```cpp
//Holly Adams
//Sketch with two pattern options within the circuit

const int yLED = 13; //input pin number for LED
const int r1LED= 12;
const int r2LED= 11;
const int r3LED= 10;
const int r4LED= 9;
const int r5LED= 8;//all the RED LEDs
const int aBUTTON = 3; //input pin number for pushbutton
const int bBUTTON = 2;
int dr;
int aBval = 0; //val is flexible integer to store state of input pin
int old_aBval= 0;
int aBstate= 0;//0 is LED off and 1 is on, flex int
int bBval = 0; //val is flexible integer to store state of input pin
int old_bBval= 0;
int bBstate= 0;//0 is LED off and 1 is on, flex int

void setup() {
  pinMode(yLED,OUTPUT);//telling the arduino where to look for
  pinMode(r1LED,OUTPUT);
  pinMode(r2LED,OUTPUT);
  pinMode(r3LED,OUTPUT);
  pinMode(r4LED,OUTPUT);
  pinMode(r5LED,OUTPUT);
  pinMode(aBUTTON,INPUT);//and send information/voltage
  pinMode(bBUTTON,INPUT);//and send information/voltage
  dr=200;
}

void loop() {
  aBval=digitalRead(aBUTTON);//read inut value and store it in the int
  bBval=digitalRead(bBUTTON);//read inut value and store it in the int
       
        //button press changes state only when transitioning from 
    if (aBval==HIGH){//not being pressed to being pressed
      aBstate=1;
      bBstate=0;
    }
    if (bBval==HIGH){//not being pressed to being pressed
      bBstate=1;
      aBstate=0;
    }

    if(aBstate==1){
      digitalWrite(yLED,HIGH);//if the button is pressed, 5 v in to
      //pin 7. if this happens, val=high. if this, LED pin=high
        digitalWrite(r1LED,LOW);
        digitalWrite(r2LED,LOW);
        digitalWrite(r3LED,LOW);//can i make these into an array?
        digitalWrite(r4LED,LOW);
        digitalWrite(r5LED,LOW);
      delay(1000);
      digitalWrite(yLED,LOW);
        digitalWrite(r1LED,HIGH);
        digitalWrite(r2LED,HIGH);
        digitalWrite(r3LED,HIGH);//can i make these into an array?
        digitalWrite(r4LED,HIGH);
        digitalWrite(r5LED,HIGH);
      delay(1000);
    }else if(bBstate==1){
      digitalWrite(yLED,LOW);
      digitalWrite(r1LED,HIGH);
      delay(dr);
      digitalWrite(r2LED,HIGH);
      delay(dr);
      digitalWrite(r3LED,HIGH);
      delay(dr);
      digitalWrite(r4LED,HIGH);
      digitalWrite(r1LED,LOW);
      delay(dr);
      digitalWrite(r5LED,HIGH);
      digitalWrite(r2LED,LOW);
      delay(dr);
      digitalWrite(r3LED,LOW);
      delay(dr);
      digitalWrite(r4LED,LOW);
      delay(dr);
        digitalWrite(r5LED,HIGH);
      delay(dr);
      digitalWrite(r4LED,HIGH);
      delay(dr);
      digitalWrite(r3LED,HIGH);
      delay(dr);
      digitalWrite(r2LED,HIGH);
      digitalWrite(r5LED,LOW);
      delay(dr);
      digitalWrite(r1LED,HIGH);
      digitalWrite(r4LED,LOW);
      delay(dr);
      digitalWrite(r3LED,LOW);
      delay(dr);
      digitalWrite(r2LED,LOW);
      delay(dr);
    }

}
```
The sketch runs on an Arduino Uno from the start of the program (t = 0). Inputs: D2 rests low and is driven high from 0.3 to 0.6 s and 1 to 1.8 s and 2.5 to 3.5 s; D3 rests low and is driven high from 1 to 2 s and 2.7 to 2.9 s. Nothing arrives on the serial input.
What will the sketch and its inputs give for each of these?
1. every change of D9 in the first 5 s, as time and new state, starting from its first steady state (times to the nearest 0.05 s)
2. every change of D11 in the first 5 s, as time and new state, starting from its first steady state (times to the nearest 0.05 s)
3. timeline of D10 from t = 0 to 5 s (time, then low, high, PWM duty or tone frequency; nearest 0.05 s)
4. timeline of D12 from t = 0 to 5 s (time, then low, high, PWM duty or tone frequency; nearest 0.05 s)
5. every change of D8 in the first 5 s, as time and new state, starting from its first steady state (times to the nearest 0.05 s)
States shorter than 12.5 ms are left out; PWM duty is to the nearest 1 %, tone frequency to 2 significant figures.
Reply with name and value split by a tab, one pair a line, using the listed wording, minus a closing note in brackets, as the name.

every change of D9 in the first 5 s, as time and new state, starting from its first steady state	0 s low; 0.9 s high; 1.5 s low; 1.9 s high; 2.5 s low; 3.7 s high; 4.3 s low; 4.7 s high
every change of D11 in the first 5 s, as time and new state, starting from its first steady state	0 s low; 0.5 s high; 1.1 s low; 2.3 s high; 2.9 s low; 3.3 s high; 3.9 s low
timeline of D10 from t = 0 to 5 s	0 s low; 0.7 s high; 1.3 s low; 2.1 s high; 2.7 s low; 3.5 s high; 4.1 s low; 4.9 s high
timeline of D12 from t = 0 to 5 s	0 s low; 0.3 s high; 0.9 s low; 2.5 s high; 3.7 s low
every change of D8 in the first 5 s, as time and new state, starting from its first steady state	0 s low; 1.1 s high; 2.3 s low; 3.9 s high
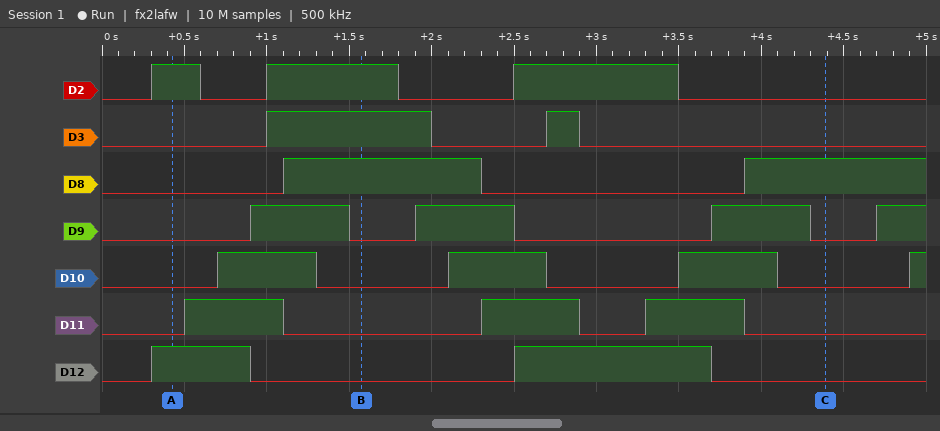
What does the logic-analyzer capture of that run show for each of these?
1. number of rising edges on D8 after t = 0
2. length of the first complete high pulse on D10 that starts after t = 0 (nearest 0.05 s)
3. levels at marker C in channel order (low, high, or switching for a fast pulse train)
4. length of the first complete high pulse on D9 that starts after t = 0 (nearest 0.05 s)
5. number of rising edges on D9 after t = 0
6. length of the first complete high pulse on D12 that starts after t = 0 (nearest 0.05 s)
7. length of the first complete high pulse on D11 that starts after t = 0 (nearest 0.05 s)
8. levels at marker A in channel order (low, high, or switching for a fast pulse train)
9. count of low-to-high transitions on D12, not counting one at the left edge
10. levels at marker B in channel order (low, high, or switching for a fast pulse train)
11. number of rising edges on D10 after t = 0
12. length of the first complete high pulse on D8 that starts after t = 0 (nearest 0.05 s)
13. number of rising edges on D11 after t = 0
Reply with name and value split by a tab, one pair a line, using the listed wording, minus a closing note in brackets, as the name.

number of rising edges on D8 after t = 0	2
length of the first complete high pulse on D10 that starts after t = 0	0.60 s
levels at marker C in channel order	D2 low, D3 low, D8 high, D9 low, D10 low, D11 low, D12 low
length of the first complete high pulse on D9 that starts after t = 0	0.60 s
number of rising edges on D9 after t = 0	4
length of the first complete high pulse on D12 that starts after t = 0	0.60 s
length of the first complete high pulse on D11 that starts after t = 0	0.60 s
levels at marker A in channel order	D2 high, D3 low, D8 low, D9 low, D10 low, D11 low, D12 high
count of low-to-high transitions on D12, not counting one at the left edge	2
levels at marker B in channel order	D2 high, D3 high, D8 high, D9 low, D10 low, D11 low, D12 low
number of rising edges on D10 after t = 0	4
length of the first complete high pulse on D8 that starts after t = 0	1.20 s
number of rising edges on D11 after t = 0	3
